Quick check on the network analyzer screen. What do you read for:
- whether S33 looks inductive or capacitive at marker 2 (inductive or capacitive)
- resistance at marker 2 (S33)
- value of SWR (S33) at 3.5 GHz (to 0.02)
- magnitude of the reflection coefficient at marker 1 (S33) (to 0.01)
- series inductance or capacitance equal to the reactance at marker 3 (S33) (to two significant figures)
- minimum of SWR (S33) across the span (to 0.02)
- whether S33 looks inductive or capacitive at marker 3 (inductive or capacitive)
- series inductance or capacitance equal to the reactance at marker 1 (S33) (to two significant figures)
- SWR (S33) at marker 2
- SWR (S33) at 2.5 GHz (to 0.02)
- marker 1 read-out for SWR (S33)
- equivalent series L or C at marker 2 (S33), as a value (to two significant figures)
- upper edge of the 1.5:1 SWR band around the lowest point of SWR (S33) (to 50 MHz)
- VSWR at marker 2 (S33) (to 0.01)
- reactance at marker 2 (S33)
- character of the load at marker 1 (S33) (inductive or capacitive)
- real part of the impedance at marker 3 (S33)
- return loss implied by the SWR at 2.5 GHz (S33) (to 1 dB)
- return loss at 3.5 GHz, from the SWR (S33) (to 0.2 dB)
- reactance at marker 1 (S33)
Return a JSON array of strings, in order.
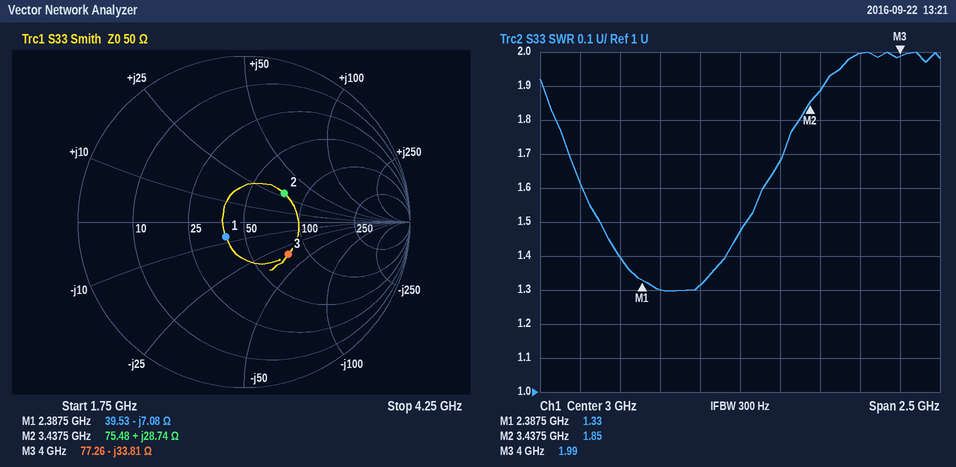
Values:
["inductive", "75.48 Ω", "1.88", "0.14", "1.2 pF", "1.30", "capacitive", "9.4 pF", "1.85", "1.30", "1.33", "1.3 nH", "3.05 GHz", "1.85", "+28.74 Ω", "capacitive", "77.26 Ω", "18 dB", "10.2 dB", "-7.08 Ω"]
